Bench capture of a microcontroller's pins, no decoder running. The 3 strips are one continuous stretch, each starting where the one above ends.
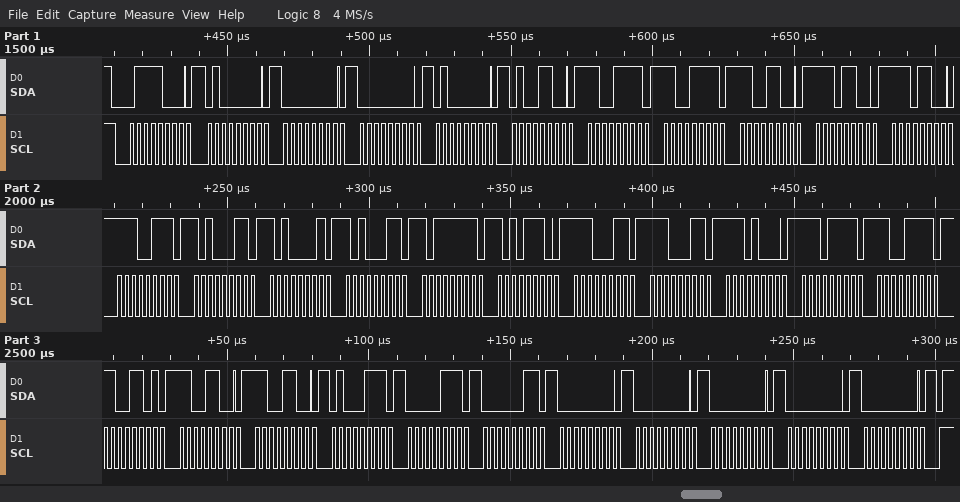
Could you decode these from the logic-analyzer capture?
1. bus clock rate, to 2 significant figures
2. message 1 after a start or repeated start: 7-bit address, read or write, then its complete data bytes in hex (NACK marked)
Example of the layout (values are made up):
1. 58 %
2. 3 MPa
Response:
1. 400 kHz
2. 0x3C write: 40 00 00 40 4C CF CF CC EC EC E7 A3 A1 A3 BF AE E3 E3 E8 EF CF CD CC CC 47 07 03 00 00 00 00 00
